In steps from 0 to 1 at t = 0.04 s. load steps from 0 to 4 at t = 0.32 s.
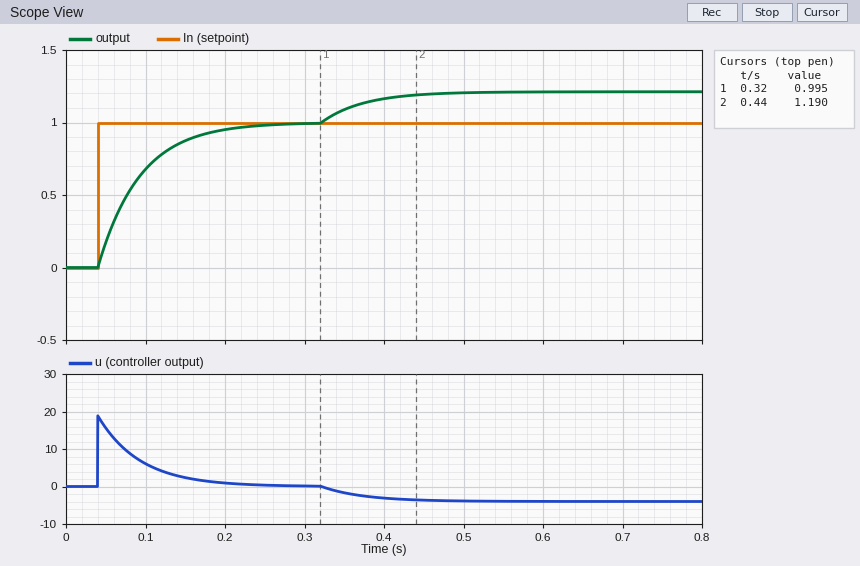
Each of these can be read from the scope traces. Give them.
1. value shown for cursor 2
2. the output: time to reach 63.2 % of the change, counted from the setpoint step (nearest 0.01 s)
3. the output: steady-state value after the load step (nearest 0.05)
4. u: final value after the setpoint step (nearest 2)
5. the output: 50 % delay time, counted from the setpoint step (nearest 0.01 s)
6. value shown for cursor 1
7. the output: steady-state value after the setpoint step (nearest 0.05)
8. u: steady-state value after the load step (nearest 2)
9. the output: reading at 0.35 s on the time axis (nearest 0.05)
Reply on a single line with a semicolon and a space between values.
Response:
1.190; 0.05 s; 1.20; 0; 0.04 s; 0.995; 1.00; -4; 1.10
